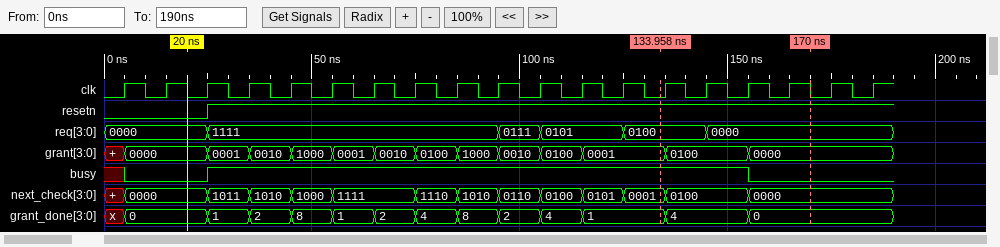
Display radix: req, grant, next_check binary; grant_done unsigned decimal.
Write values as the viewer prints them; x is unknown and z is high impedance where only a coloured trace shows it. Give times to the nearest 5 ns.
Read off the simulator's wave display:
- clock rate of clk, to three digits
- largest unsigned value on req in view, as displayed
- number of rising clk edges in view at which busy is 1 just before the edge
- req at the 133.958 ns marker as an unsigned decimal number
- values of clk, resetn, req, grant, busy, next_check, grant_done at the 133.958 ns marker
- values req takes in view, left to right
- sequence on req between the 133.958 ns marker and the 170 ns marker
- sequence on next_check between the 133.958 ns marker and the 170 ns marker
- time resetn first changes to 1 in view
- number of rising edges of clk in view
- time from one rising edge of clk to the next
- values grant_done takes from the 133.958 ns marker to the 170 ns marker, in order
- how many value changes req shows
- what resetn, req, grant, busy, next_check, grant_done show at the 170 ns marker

100 MHz
1111
13
4
clk=0, resetn=1, req=0100, grant=0001, busy=1, next_check=0001, grant_done=1
0000, 1111, 0111, 0101, 0100, 0000
0100, 0000
0001, 0100, 0000
25 ns
19
10 ns
1, 4, 0
5
resetn=1, req=0000, grant=0000, busy=0, next_check=0000, grant_done=0
